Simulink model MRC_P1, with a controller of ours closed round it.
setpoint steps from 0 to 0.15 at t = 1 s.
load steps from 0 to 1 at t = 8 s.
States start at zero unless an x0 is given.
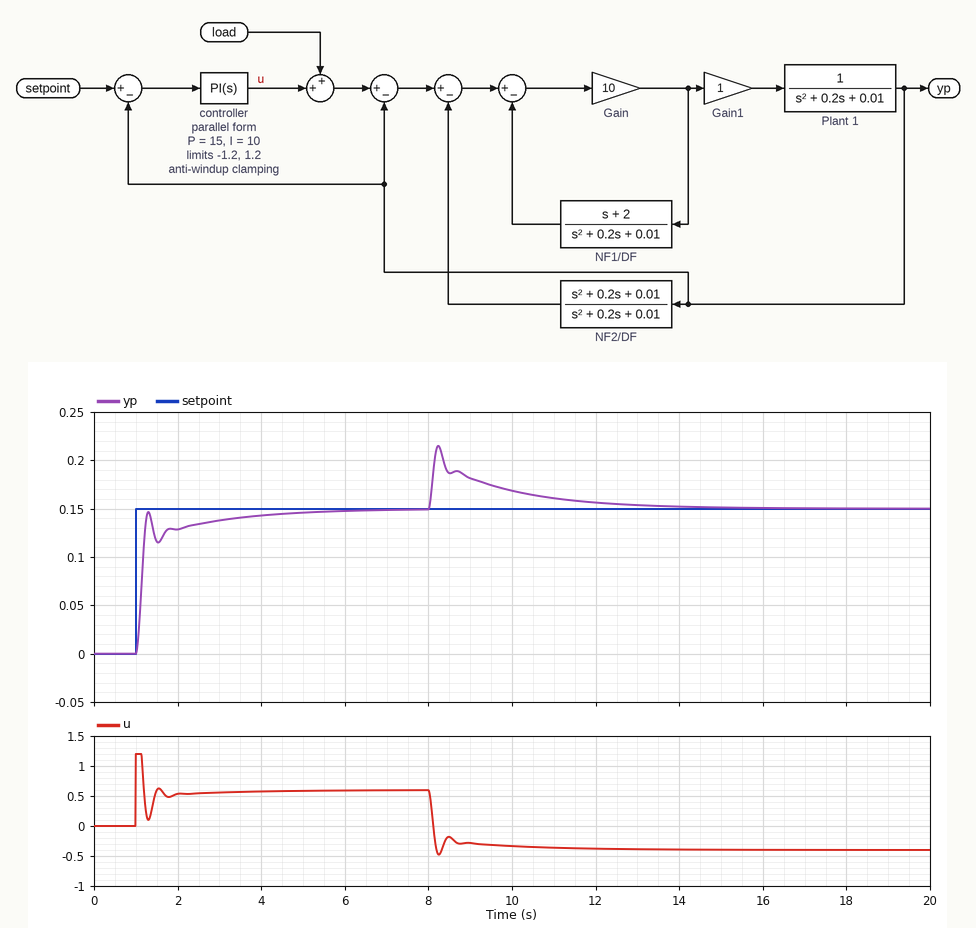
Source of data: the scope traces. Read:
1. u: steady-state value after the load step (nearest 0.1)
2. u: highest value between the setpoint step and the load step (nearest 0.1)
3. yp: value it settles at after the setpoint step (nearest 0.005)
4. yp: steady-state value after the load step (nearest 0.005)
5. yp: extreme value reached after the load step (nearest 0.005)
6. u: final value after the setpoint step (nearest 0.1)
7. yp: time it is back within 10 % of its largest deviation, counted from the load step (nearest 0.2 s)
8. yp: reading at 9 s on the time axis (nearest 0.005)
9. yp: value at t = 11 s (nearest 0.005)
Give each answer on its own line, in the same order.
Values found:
-0.4
1.2
0.150
0.150
0.215
0.6
4.0 s
0.180
0.160
